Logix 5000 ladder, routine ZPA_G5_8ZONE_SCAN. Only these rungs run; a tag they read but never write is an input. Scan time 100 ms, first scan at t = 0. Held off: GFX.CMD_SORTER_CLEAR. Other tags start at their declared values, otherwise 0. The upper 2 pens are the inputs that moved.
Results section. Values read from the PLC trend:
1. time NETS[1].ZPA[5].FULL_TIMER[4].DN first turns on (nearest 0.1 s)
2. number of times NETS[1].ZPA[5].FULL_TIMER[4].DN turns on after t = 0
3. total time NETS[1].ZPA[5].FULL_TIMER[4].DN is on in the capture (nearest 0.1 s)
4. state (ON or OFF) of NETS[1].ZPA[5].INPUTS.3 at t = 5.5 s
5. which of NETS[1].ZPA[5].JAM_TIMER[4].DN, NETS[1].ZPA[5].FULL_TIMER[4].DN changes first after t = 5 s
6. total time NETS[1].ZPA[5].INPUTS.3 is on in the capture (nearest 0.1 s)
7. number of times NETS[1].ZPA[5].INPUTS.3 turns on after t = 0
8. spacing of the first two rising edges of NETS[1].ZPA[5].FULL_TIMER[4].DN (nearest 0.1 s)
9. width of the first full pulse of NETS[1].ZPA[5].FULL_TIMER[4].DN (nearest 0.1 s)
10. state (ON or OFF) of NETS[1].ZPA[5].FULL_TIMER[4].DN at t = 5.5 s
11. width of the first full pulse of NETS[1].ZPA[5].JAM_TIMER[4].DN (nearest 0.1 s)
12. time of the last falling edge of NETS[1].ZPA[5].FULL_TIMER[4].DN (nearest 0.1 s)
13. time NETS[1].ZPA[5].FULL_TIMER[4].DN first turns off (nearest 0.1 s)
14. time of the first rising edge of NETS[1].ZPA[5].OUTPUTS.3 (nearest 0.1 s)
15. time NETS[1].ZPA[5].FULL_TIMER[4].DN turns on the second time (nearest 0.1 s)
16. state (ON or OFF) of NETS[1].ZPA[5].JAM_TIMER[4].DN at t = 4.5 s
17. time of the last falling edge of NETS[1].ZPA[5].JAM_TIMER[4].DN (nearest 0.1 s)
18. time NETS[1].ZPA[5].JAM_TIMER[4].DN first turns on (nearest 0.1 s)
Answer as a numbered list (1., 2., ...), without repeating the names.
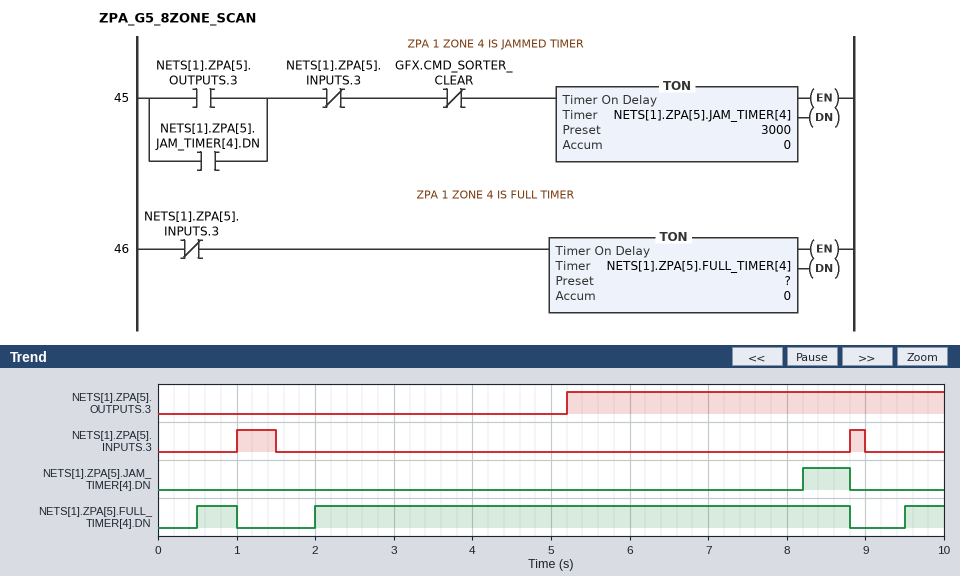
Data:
1. 0.5 s
2. 3
3. 7.8 s
4. OFF
5. NETS[1].ZPA[5].JAM_TIMER[4].DN
6. 0.7 s
7. 2
8. 1.5 s
9. 0.5 s
10. ON
11. 0.6 s
12. 8.8 s
13. 1.0 s
14. 5.2 s
15. 2.0 s
16. OFF
17. 8.8 s
18. 8.2 s
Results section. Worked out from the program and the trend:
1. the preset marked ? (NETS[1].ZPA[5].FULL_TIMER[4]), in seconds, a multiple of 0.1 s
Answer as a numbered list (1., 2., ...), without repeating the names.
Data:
1. 0.5 s
